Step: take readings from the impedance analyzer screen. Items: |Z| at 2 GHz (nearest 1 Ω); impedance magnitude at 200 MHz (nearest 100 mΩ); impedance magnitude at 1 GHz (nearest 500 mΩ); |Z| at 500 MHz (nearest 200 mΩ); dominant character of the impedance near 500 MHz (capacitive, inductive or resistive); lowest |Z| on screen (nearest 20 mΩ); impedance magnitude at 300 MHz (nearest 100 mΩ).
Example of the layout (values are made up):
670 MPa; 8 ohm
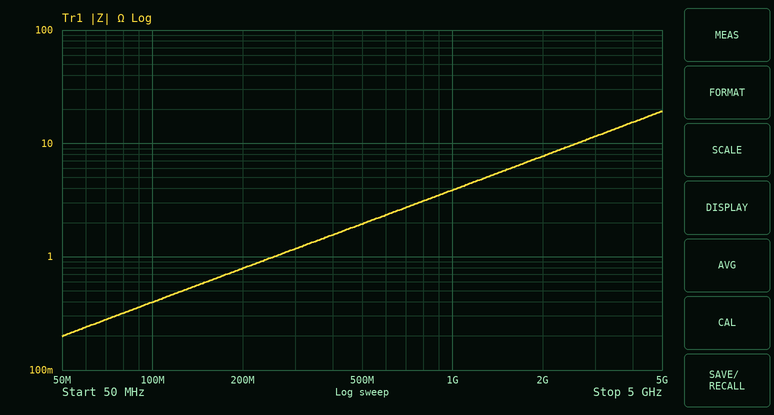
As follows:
8 Ω; 800 mΩ; 4.0 Ω; 2.0 Ω; inductive; 200 mΩ; 1.2 Ω
